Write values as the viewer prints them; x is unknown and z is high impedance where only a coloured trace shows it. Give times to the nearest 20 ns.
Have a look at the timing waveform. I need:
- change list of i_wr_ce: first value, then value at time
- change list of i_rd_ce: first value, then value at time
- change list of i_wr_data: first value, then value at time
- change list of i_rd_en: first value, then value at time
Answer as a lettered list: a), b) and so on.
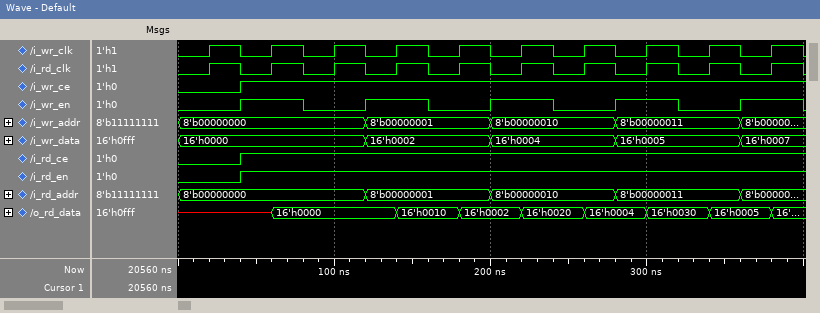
a) 0, 1 at 40 ns
b) 0, 1 at 40 ns
c) 16'h0000, 16'h0002 at 120 ns, 16'h0004 at 200 ns, 16'h0005 at 280 ns, 16'h0007 at 360 ns
d) 0, 1 at 40 ns
